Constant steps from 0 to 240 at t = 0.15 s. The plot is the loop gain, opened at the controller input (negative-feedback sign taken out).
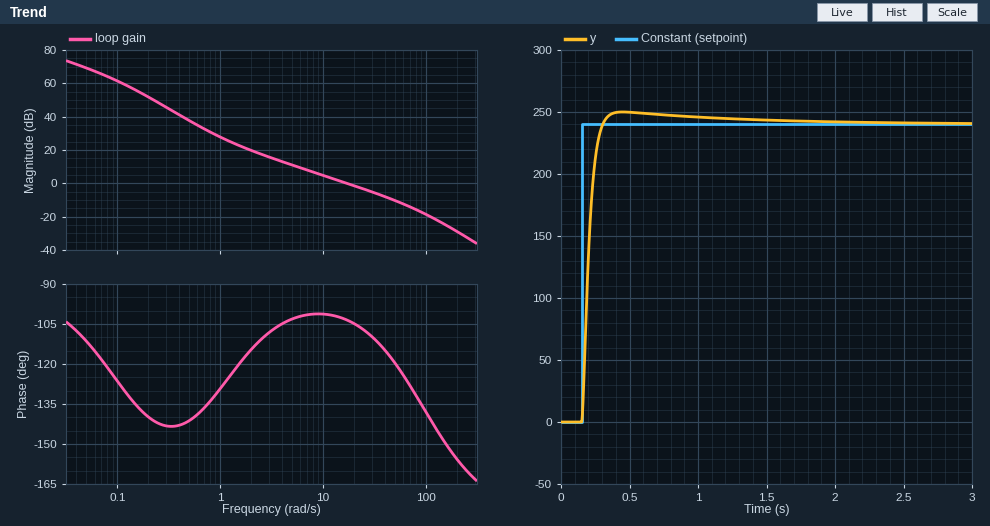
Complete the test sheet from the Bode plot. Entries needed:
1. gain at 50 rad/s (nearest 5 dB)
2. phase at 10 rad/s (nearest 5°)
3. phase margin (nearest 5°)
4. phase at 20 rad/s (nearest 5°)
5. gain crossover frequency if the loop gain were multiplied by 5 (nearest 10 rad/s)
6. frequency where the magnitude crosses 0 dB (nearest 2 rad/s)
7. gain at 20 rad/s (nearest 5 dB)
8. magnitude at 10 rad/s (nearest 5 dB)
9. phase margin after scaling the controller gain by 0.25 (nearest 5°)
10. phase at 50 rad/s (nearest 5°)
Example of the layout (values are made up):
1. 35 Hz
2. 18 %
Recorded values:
1. -10 dB
2. -100°
3. 75°
4. -105°
5. 70 rad/s
6. 18 rad/s
7. 0 dB
8. 5 dB
9. 75°
10. -120°
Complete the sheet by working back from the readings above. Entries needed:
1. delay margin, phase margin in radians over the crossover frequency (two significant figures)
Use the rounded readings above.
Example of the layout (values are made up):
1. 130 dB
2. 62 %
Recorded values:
1. 0.073 s
